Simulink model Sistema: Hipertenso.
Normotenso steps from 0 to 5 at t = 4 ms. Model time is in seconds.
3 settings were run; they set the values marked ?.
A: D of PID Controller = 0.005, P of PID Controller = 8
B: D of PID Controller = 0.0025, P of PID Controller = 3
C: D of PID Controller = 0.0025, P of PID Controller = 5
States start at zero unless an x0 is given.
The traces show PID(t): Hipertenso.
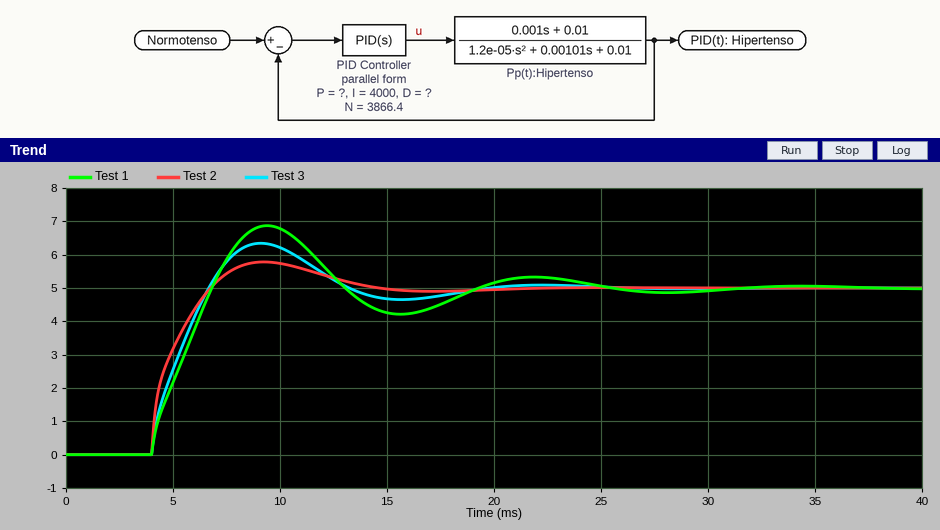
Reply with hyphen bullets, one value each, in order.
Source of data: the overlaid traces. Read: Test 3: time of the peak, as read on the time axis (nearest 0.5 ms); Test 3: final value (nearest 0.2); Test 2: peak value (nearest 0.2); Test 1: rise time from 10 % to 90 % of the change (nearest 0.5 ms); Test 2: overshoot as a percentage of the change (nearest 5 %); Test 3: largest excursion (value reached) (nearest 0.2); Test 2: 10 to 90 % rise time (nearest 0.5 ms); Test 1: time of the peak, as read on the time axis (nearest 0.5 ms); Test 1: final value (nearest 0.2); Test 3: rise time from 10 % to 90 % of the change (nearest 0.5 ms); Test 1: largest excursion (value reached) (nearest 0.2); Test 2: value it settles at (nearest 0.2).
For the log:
- 9.0 ms
- 5.0
- 5.8
- 2.5 ms
- 15 %
- 6.4
- 2.0 ms
- 9.5 ms
- 5.0
- 2.0 ms
- 6.8
- 5.0
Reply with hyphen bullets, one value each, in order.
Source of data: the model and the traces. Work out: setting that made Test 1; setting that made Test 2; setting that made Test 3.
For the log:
- B
- A
- C
